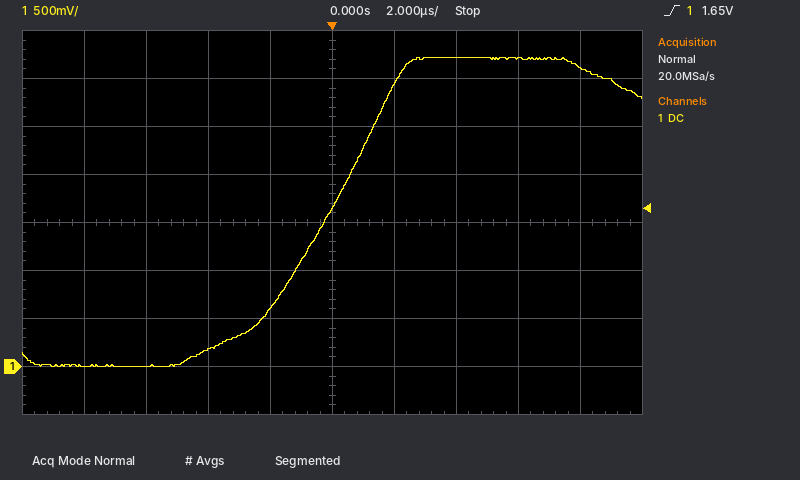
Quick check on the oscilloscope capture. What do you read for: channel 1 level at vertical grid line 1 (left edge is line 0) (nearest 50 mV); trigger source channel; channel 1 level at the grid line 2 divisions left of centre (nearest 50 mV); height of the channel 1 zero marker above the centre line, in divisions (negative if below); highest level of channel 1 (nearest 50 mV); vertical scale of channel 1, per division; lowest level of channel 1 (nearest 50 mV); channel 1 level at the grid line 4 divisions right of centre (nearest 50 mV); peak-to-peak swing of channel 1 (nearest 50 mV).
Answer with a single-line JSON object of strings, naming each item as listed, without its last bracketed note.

{"channel 1 level at vertical grid line 1 (left edge is line 0)": "0 mV", "trigger source channel": "channel 1", "channel 1 level at the grid line 2 divisions left of centre": "200 mV", "height of the channel 1 zero marker above the centre line, in divisions": "-3.0 div", "highest level of channel 1": "3.20 V", "vertical scale of channel 1, per division": "500 mV", "lowest level of channel 1": "0 mV", "channel 1 level at the grid line 4 divisions right of centre": "3.10 V", "peak-to-peak swing of channel 1": "3.20 V"}
